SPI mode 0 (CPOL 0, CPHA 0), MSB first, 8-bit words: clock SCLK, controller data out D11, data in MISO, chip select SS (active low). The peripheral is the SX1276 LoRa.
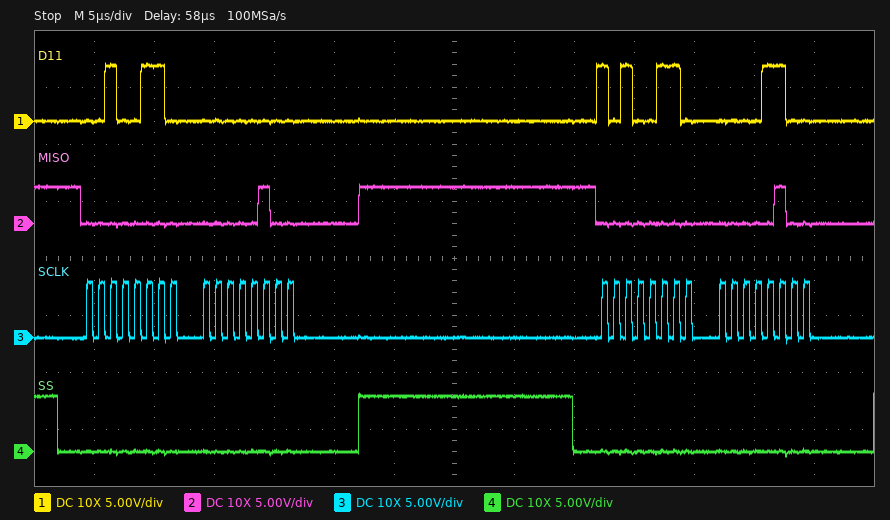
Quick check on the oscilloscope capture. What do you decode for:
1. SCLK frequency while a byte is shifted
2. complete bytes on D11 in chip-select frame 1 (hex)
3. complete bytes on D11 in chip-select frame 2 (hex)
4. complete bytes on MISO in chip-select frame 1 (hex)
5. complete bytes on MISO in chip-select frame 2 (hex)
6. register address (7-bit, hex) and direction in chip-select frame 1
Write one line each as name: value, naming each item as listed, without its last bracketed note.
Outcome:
SCLK frequency while a byte is shifted: 1 MHz
complete bytes on D11 in chip-select frame 1: 26 00
complete bytes on D11 in chip-select frame 2: A6 0C
complete bytes on MISO in chip-select frame 1: 00 04
complete bytes on MISO in chip-select frame 2: 00 04
register address (7-bit, hex) and direction in chip-select frame 1: 0x26 read
